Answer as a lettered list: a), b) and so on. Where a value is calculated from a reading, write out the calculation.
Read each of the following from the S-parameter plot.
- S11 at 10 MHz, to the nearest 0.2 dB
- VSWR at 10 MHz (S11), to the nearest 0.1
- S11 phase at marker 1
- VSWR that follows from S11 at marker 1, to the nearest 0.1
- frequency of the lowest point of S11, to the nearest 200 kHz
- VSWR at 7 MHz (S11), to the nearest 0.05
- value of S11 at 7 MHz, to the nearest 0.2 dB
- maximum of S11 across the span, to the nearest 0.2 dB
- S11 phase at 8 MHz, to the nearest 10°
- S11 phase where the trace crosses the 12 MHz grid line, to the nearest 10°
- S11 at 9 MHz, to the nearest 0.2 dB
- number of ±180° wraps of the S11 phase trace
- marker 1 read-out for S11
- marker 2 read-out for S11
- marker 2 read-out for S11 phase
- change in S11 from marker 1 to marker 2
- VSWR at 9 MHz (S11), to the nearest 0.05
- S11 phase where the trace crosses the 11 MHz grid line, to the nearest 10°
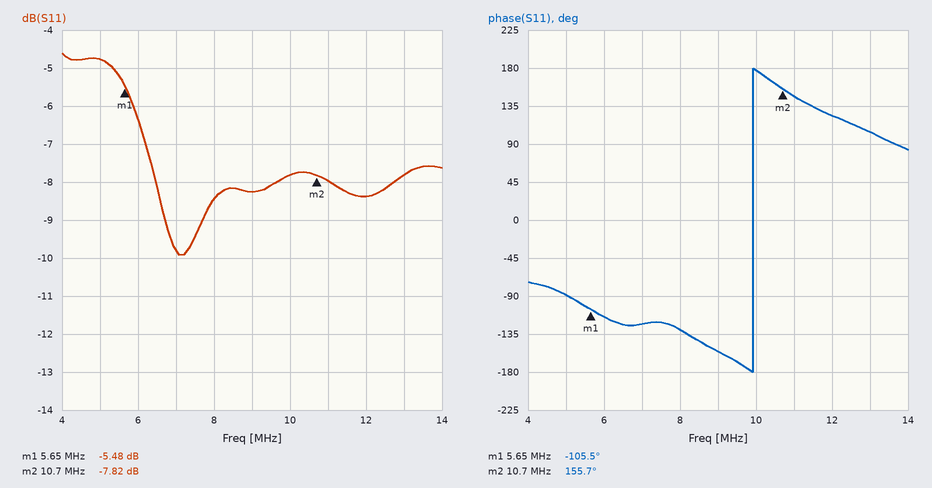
a) -7.8 dB
b) |Γ| = 10^(-7.8/20) = 0.4074; VSWR = (1 + 0.4074)/(1 − 0.4074) ≈ 2.4
c) -105.5°
d) (1 + 0.5321)/(1 − 0.5321) ≈ 3.3
e) 7.0 MHz
f) |Γ| = 10^(-9.8/20) = 0.3236; VSWR = (1 + 0.3236)/(1 − 0.3236) ≈ 1.96, so 1.95 to the nearest 0.05
g) -9.8 dB
h) -4.6 dB
i) -130°
j) 120°
k) -8.2 dB
l) 1
m) -5.48 dB
n) -7.82 dB
o) 155.7°
p) -7.82 − (-5.48) = -2.34 dB
q) |Γ| = 10^(-8.2/20) = 0.3890; VSWR = (1 + 0.3890)/(1 − 0.3890) ≈ 2.27, so 2.25 to the nearest 0.05
r) 150°
